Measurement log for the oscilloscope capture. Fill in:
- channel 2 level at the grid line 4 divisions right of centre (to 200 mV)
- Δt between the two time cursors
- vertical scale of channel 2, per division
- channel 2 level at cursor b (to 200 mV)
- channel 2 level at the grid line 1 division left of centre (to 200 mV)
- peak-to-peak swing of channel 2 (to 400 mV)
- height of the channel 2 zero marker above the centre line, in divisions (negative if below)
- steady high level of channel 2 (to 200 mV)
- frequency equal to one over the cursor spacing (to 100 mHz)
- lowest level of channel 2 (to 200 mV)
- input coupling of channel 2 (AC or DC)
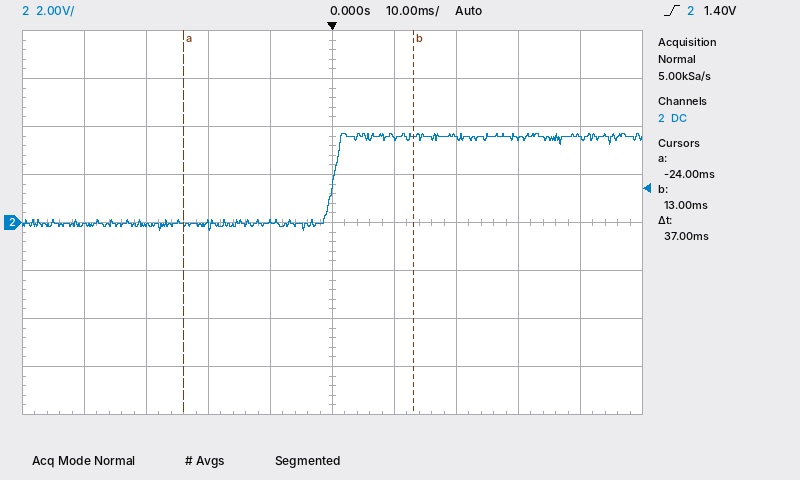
3.6 V
37 ms
2 V
3.6 V
0.0 V
4.0 V
0.0 div
3.6 V
27.0 Hz
-400 mV
DC
